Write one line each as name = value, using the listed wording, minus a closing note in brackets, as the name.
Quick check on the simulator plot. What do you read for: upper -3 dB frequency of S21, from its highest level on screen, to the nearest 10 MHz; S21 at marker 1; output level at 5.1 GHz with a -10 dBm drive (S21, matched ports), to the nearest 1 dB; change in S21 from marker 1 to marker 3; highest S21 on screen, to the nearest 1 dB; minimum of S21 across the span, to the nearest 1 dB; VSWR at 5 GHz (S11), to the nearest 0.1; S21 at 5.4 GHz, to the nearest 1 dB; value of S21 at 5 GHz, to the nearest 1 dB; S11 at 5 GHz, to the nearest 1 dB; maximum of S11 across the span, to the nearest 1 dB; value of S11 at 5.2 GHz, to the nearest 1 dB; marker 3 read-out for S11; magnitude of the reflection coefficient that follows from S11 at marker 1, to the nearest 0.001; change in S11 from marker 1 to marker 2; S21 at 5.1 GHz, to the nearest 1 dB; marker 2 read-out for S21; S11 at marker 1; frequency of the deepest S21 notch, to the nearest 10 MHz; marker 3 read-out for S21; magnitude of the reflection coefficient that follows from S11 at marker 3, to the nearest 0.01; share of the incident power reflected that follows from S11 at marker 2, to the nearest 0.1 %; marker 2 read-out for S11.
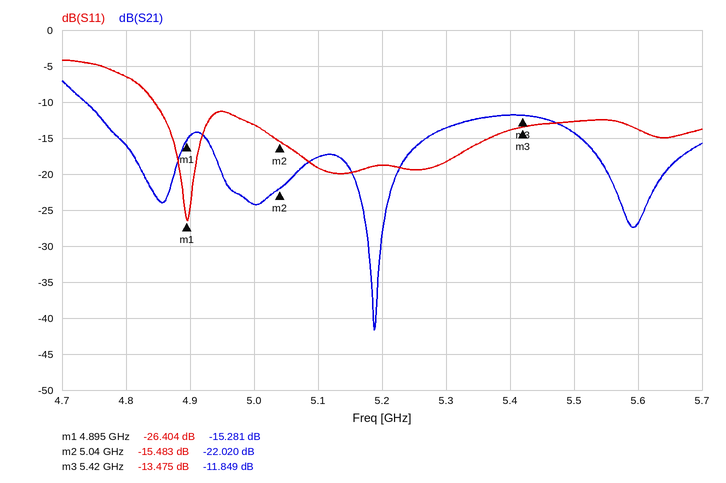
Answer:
upper -3 dB frequency of S21, from its highest level on screen, to the nearest 10 MHz = 4.74 GHz
S21 at marker 1 = -15.281 dB
output level at 5.1 GHz with a -10 dBm drive (S21, matched ports), to the nearest 1 dB = -28 dBm
change in S21 from marker 1 to marker 3 = 3.432 dB
highest S21 on screen, to the nearest 1 dB = -7 dB
minimum of S21 across the span, to the nearest 1 dB = -42 dB
VSWR at 5 GHz (S11), to the nearest 0.1 = 1.6
S21 at 5.4 GHz, to the nearest 1 dB = -12 dB
value of S21 at 5 GHz, to the nearest 1 dB = -24 dB
S11 at 5 GHz, to the nearest 1 dB = -13 dB
maximum of S11 across the span, to the nearest 1 dB = -4 dB
value of S11 at 5.2 GHz, to the nearest 1 dB = -19 dB
marker 3 read-out for S11 = -13.475 dB
magnitude of the reflection coefficient that follows from S11 at marker 1, to the nearest 0.001 = 0.048
change in S11 from marker 1 to marker 2 = 10.921 dB
S21 at 5.1 GHz, to the nearest 1 dB = -18 dB
marker 2 read-out for S21 = -22.020 dB
S11 at marker 1 = -26.404 dB
frequency of the deepest S21 notch, to the nearest 10 MHz = 5.19 GHz
marker 3 read-out for S21 = -11.849 dB
magnitude of the reflection coefficient that follows from S11 at marker 3, to the nearest 0.01 = 0.21
share of the incident power reflected that follows from S11 at marker 2, to the nearest 0.1 % = 2.8 %
marker 2 read-out for S11 = -15.483 dB
